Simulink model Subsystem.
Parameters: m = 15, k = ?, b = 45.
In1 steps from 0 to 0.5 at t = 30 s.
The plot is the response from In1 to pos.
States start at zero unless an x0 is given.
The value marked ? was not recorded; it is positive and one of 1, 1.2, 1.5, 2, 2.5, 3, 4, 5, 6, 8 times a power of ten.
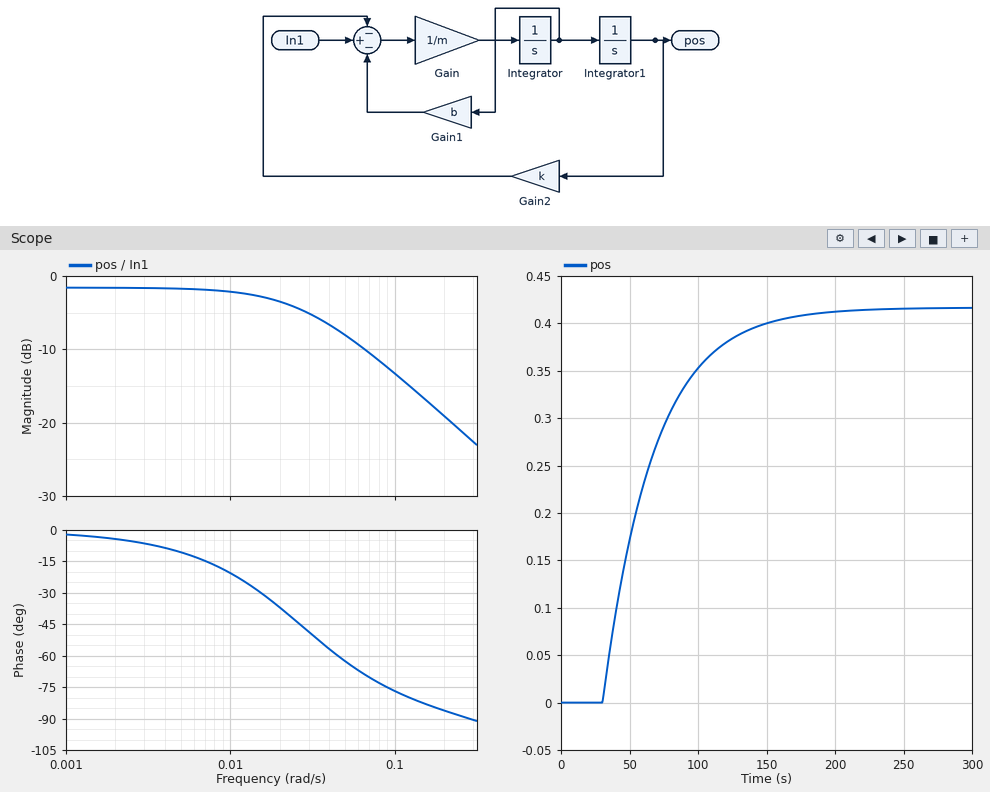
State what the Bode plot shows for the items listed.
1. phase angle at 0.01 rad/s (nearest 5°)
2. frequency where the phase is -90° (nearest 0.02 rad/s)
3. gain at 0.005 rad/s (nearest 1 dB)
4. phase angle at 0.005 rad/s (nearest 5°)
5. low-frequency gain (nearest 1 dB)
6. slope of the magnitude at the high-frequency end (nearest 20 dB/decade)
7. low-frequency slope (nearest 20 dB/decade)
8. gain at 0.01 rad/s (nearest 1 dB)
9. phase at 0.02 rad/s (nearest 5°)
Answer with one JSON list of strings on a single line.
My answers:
["-20°", "0.28 rad/s", "-2 dB", "-10°", "-2 dB", "-20 dB/decade", "0 dB/decade", "-2 dB", "-35°"]
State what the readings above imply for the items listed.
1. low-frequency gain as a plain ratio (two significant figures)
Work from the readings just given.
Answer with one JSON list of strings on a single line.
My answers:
["0.79"]
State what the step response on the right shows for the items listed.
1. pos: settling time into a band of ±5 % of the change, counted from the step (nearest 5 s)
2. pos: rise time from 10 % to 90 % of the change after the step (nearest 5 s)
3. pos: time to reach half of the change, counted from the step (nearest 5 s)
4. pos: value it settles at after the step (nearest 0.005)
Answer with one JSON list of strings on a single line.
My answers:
["110 s", "80 s", "25 s", "0.415"]
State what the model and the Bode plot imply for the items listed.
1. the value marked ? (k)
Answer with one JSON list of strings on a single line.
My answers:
["1.2"]
